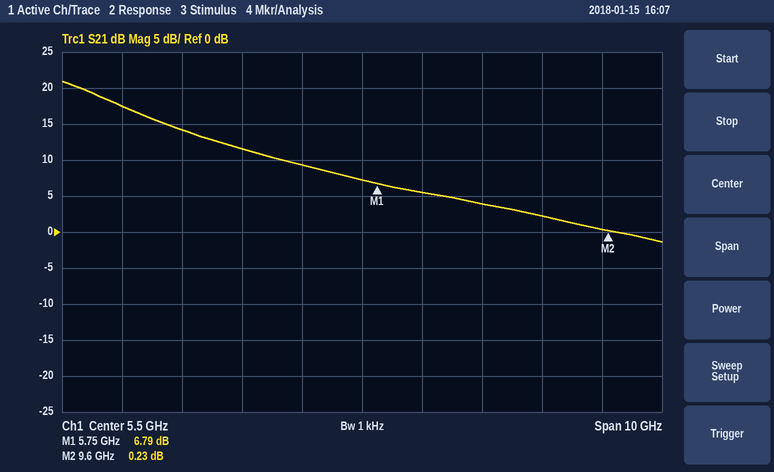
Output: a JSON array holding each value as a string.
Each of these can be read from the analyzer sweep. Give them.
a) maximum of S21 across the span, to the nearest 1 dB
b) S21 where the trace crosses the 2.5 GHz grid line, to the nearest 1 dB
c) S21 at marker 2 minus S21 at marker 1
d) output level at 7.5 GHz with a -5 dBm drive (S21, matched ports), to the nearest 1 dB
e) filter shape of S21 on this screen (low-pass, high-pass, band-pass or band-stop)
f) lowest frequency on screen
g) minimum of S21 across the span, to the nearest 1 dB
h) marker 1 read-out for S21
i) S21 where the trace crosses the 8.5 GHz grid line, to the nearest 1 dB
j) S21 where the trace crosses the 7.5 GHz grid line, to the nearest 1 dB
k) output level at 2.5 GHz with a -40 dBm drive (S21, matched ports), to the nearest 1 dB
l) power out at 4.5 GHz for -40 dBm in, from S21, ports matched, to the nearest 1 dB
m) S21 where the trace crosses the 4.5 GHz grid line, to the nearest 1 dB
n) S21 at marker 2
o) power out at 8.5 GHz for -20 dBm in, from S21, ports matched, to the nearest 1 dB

["21 dB", "14 dB", "-6.56 dB", "-1 dBm", "low-pass", "500 MHz", "-1 dB", "6.79 dB", "2 dB", "4 dB", "-26 dBm", "-31 dBm", "9 dB", "0.23 dB", "-18 dBm"]
